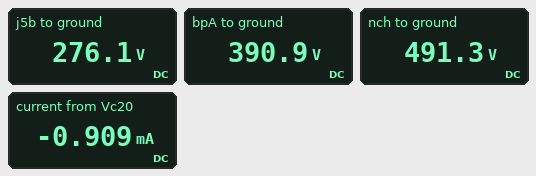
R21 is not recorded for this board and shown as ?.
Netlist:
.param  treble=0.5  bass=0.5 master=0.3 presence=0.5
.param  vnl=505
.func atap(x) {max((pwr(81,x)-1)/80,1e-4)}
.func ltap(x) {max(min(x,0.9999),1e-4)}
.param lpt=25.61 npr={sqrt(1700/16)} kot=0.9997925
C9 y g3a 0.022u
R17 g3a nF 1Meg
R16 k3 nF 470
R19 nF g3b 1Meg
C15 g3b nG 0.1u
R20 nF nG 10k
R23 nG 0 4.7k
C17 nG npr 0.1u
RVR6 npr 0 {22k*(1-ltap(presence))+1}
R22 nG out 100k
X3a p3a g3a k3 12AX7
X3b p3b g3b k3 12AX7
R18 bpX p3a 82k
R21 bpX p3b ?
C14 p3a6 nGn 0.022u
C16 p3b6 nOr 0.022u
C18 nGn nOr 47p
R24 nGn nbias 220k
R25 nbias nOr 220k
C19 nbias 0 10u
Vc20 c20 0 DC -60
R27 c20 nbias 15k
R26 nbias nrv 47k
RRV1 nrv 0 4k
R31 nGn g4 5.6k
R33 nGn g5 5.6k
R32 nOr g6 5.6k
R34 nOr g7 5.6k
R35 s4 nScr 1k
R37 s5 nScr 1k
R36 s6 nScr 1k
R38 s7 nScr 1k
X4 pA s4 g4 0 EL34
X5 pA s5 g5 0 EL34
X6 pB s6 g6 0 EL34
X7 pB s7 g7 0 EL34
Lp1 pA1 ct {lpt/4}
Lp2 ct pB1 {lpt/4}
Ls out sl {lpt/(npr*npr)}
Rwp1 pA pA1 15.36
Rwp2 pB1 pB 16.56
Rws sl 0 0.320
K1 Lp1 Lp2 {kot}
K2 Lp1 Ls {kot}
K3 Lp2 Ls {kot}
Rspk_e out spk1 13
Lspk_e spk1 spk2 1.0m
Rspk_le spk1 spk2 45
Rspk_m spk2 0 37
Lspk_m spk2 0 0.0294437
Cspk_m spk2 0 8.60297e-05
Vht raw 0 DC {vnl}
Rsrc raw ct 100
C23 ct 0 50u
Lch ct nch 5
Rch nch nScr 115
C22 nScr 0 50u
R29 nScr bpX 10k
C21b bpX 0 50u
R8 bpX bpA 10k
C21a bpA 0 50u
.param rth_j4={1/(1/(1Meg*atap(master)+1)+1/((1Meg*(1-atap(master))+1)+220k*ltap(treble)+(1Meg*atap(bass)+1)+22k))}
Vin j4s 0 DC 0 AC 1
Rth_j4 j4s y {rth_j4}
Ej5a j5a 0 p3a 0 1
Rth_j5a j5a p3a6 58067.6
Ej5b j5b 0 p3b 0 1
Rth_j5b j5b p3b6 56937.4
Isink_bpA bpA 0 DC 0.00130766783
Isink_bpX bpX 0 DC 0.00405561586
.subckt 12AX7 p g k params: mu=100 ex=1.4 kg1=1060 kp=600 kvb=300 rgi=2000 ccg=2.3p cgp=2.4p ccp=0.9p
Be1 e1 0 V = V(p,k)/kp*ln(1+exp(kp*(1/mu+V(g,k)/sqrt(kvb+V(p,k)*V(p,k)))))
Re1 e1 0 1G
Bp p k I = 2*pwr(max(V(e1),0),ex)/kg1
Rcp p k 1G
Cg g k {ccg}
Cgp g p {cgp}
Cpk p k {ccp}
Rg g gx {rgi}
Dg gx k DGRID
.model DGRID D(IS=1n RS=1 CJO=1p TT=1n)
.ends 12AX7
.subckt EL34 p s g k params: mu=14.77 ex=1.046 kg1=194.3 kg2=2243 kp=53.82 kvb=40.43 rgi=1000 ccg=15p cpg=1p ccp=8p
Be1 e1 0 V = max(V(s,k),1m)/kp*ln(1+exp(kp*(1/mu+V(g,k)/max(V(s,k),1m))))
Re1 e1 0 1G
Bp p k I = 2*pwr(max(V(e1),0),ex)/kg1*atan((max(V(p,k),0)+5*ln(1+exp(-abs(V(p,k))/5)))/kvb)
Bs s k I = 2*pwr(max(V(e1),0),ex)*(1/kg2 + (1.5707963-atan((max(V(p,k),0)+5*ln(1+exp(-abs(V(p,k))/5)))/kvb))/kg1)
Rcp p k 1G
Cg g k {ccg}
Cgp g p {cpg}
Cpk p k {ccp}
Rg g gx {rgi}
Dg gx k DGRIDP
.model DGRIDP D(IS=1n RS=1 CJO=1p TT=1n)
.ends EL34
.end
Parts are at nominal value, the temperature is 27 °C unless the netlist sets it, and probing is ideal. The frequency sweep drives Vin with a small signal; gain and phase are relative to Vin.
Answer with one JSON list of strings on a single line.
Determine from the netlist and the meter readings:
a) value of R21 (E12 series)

["82 kΩ"]
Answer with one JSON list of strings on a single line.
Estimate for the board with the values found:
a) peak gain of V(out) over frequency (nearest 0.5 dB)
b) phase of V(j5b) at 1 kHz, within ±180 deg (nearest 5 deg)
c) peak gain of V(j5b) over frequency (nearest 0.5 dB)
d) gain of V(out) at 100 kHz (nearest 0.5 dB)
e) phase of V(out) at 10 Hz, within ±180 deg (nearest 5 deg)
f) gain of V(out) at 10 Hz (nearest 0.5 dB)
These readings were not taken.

["27.0 dB", "-5 deg", "28.0 dB", "20.0 dB", "130 deg", "12.5 dB"]
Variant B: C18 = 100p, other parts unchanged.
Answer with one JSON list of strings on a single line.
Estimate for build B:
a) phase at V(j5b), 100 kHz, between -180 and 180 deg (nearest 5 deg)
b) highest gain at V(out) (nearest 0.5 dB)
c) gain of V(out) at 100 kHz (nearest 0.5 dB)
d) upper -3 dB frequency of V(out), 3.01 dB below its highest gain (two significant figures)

["-55 deg", "26.0 dB", "15.0 dB", "56 kHz"]
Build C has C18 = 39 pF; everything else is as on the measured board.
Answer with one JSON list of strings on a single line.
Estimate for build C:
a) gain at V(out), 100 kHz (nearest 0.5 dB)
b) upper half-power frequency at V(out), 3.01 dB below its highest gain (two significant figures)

["21.0 dB", "82 kHz"]
